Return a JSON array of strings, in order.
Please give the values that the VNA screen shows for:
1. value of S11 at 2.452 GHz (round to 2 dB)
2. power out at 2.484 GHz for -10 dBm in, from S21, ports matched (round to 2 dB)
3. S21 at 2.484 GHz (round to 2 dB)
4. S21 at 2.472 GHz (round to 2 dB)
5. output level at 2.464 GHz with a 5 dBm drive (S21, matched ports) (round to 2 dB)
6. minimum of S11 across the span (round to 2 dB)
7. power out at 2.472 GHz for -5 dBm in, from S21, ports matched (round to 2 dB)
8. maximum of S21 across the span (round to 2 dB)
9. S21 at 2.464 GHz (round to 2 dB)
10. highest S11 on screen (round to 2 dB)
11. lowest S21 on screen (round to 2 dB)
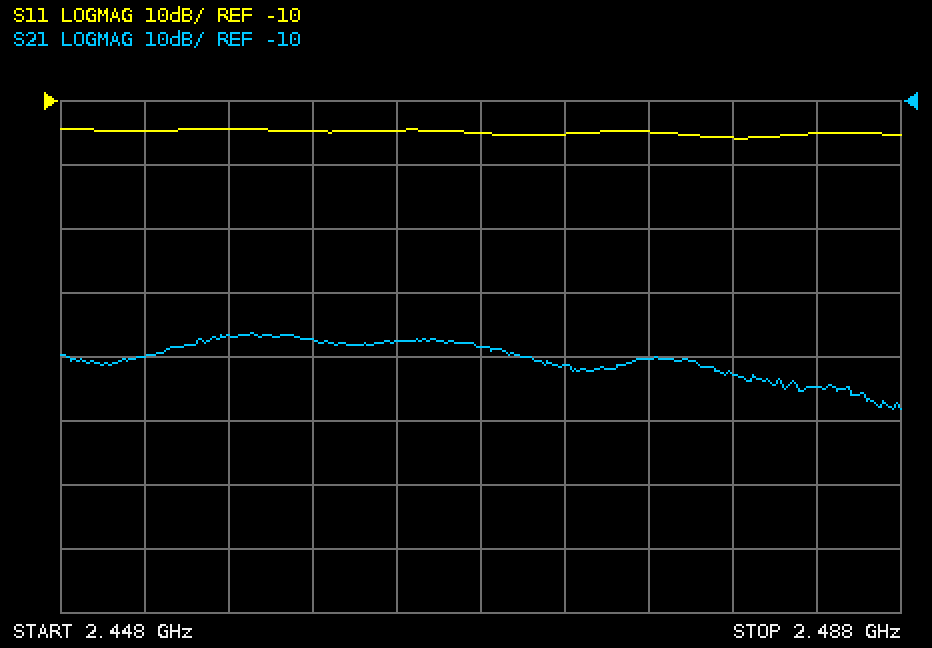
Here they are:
["-14 dB", "-64 dBm", "-54 dB", "-52 dB", "-42 dBm", "-16 dB", "-56 dBm", "-46 dB", "-48 dB", "-14 dB", "-58 dB"]
